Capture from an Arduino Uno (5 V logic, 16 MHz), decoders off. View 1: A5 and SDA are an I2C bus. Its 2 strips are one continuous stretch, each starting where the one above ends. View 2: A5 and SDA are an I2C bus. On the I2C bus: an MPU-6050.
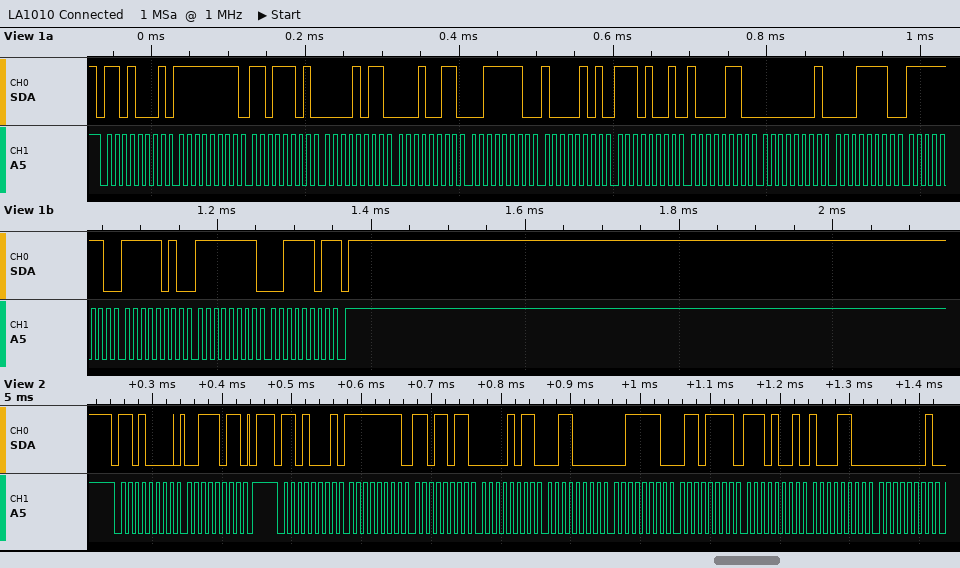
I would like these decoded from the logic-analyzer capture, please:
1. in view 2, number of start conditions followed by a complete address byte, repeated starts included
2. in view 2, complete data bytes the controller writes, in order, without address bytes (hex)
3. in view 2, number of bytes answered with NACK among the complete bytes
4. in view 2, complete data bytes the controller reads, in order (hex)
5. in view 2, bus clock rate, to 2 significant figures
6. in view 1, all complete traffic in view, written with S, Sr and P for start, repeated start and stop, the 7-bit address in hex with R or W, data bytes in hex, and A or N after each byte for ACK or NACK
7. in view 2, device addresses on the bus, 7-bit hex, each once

2
3B
0
FF DB 0B 30 3E 6F E9 8C 01
100 kHz
S 68R A FF A DD A 0B A 13 A 3E A 85 A E9 A 86 A 01 A 1E A FE A FA A FF A 3D N P
0x68
